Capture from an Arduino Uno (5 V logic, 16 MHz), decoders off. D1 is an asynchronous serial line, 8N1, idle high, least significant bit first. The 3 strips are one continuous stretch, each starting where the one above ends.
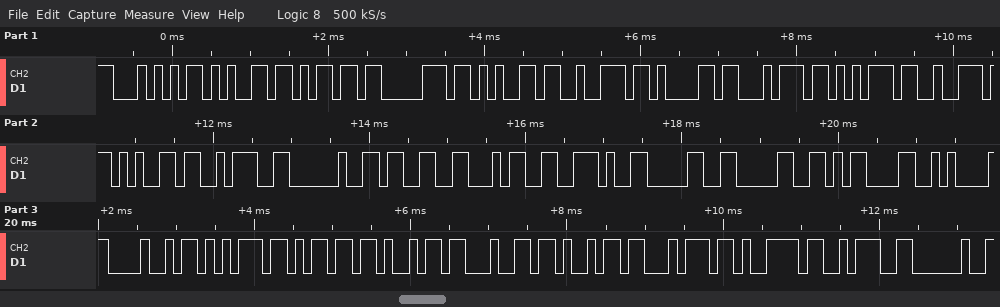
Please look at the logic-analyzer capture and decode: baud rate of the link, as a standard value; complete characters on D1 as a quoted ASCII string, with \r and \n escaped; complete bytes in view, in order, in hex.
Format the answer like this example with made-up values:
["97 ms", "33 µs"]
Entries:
["9600 baud", "\"Temperature: 34.00\\r\\nHumidity: \"", "0x54 0x65 0x6D 0x70 0x65 0x72 0x61 0x74 0x75 0x72 0x65 0x3A 0x20 0x33 0x34 0x2E 0x30 0x30 0x0D 0x0A 0x48 0x75 0x6D 0x69 0x64 0x69 0x74 0x79 0x3A 0x20"]
